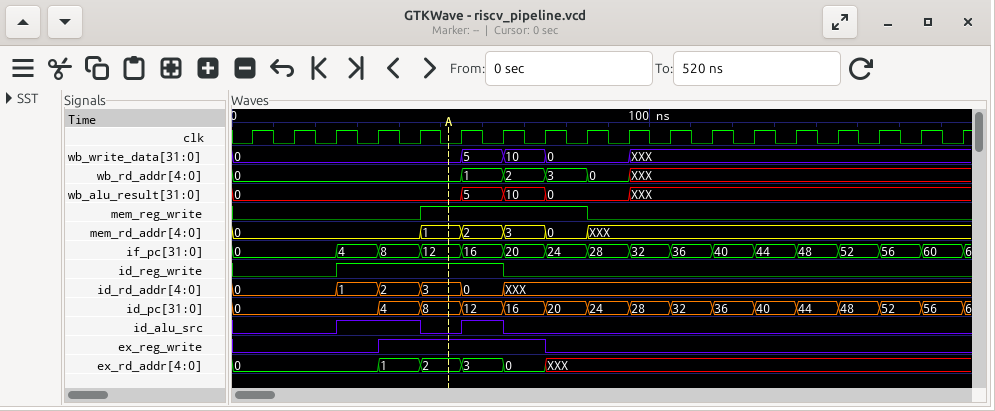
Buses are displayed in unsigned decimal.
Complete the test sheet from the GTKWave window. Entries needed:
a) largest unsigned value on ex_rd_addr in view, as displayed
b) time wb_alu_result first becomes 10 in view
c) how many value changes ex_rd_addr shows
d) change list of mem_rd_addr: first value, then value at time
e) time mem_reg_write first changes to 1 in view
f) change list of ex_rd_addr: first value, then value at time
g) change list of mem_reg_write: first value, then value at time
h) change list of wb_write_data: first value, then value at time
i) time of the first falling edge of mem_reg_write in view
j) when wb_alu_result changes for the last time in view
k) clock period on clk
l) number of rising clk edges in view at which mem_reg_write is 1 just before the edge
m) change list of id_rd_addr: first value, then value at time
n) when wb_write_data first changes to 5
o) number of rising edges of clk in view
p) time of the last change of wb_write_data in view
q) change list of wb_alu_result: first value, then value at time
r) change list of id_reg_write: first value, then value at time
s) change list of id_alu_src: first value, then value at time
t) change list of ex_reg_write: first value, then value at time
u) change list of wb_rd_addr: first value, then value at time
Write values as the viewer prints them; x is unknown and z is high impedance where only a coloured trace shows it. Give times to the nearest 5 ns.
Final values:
3
65 ns
5
0, 1 at 45 ns, 2 at 55 ns, 3 at 65 ns, 0 at 75 ns, XXX at 85 ns
45 ns
0, 1 at 35 ns, 2 at 45 ns, 3 at 55 ns, 0 at 65 ns, XXX at 75 ns
0, 1 at 45 ns, 0 at 85 ns
0, 5 at 55 ns, 10 at 65 ns, 0 at 75 ns, XXX at 95 ns
85 ns
95 ns
10 ns
4
0, 1 at 25 ns, 2 at 35 ns, 3 at 45 ns, 0 at 55 ns, XXX at 65 ns
55 ns
18
95 ns
0, 5 at 55 ns, 10 at 65 ns, 0 at 75 ns, XXX at 95 ns
0, 1 at 25 ns, 0 at 65 ns
0, 1 at 25 ns, 0 at 45 ns, 1 at 55 ns, 0 at 65 ns
0, 1 at 35 ns, 0 at 75 ns
0, 1 at 55 ns, 2 at 65 ns, 3 at 75 ns, 0 at 85 ns, XXX at 95 ns
